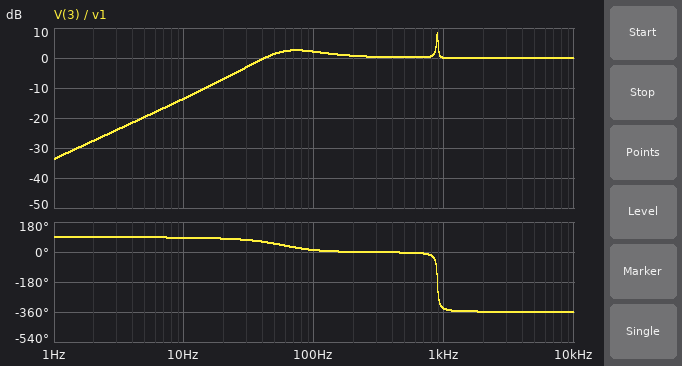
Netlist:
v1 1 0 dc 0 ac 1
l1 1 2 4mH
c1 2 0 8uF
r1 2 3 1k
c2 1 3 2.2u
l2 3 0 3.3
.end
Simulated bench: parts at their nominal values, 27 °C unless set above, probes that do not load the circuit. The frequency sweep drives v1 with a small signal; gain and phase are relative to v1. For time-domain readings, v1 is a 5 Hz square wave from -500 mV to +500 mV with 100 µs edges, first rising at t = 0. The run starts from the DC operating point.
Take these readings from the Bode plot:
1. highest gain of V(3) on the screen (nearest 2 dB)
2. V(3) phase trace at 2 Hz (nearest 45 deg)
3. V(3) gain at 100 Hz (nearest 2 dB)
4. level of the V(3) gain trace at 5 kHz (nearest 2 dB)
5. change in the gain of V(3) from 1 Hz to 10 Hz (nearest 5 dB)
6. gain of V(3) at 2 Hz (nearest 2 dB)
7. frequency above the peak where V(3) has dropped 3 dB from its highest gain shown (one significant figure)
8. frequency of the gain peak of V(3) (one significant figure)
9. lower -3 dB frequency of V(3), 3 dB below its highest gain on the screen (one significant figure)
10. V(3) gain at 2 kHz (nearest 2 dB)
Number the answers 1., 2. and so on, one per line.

1. 8 dB
2. 90 deg
3. 2 dB
4. 0 dB
5. 20 dB
6. -28 dB
7. 900 Hz
8. 900 Hz
9. 900 Hz
10. 0 dB
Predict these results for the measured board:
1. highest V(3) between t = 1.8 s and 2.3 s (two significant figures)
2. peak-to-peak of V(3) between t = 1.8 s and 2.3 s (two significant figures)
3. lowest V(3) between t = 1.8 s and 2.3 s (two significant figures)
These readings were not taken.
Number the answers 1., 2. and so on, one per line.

1. 1.0 V
2. 2.1 V
3. -1.0 V
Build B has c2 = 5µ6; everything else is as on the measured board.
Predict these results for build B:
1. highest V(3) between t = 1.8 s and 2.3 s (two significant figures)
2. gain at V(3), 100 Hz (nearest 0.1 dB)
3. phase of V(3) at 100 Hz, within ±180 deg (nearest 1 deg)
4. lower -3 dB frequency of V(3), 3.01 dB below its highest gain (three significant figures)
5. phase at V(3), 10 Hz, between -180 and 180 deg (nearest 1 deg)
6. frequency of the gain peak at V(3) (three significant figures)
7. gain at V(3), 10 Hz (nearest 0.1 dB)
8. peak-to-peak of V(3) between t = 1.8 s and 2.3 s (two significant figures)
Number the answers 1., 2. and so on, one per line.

1. 1.0 V
2. 1.2 dB
3. 2 deg
4. 29.0 Hz
5. 97 deg
6. 41.2 Hz
7. -12.7 dB
8. 2.0 V
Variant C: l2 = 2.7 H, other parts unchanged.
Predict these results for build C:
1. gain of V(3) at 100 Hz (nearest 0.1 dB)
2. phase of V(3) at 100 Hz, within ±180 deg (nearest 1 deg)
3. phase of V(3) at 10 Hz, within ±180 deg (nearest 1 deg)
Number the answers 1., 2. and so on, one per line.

1. 2.6 dB
2. 15 deg
3. 88 deg
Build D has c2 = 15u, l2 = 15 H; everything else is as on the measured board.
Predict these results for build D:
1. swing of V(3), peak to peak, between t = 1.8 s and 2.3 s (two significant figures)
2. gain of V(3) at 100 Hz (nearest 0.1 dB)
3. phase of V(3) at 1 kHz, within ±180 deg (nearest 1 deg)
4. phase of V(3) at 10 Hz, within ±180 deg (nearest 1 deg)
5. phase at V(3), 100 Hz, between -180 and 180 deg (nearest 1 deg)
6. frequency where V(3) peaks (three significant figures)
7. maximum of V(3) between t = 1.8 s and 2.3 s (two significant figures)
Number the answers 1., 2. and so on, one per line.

1. 2.0 V
2. 0.1 dB
3. 3 deg
4. 50 deg
5. 0 deg
6. 12.4 Hz
7. 990 mV
